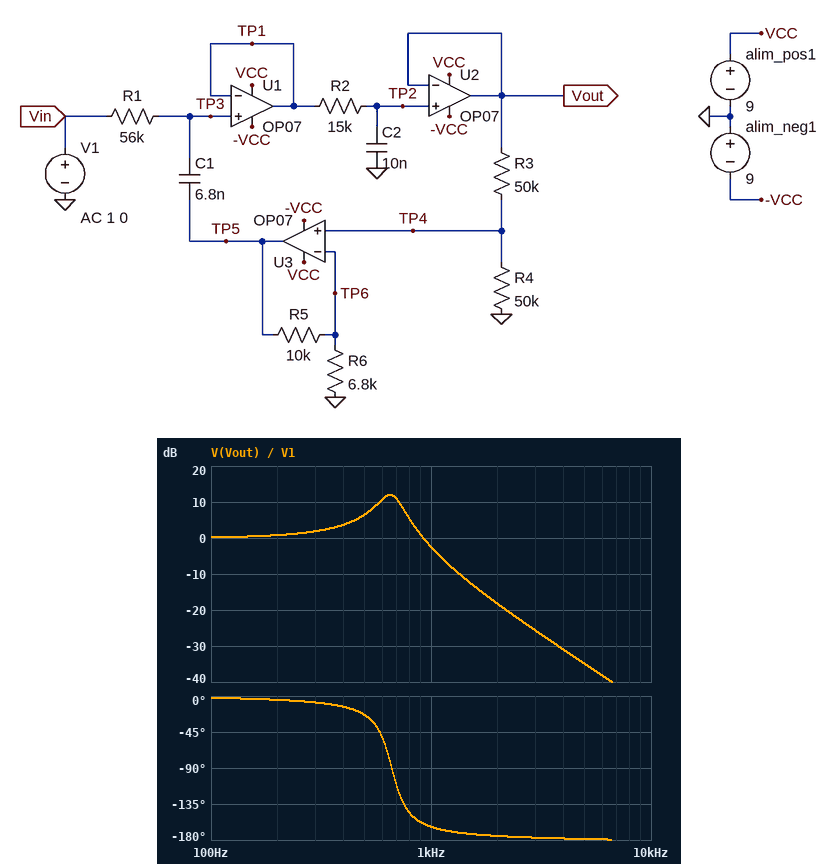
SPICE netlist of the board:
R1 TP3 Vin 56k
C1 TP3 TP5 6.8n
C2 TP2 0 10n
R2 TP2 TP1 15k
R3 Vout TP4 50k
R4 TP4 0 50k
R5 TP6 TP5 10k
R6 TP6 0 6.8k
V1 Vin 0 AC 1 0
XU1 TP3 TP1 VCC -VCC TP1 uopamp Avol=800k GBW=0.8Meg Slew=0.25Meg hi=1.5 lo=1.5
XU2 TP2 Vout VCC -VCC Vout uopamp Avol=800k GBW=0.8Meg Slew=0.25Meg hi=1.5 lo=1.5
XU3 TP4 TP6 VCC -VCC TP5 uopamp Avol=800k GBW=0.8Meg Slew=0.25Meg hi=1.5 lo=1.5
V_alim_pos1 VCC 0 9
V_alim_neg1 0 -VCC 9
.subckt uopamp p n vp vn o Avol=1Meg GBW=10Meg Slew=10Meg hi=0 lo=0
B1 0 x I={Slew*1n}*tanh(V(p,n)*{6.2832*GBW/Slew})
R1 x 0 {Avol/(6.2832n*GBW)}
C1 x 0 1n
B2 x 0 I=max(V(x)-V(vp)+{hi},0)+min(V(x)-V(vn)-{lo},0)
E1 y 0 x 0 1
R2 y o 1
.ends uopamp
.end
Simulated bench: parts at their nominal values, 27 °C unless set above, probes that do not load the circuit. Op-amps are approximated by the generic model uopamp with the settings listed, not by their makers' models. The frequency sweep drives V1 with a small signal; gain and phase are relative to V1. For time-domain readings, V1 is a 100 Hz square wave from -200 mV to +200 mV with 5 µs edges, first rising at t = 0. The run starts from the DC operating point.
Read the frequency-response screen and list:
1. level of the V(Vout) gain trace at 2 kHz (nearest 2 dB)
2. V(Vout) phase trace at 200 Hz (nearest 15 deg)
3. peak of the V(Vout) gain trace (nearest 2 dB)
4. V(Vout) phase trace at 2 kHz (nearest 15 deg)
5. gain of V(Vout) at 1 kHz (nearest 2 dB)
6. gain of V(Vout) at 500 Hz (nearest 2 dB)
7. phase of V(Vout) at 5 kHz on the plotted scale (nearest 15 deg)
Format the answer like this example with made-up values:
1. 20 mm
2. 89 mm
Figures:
1. -18 dB
2. 0 deg
3. 12 dB
4. -180 deg
5. -2 dB
6. 6 dB
7. -180 deg
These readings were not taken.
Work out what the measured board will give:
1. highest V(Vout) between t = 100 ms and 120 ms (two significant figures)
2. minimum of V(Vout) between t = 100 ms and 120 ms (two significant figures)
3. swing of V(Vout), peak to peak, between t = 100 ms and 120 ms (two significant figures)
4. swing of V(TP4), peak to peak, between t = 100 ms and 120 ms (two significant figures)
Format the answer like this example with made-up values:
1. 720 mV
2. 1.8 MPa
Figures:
1. 470 mV
2. -470 mV
3. 940 mV
4. 470 mV
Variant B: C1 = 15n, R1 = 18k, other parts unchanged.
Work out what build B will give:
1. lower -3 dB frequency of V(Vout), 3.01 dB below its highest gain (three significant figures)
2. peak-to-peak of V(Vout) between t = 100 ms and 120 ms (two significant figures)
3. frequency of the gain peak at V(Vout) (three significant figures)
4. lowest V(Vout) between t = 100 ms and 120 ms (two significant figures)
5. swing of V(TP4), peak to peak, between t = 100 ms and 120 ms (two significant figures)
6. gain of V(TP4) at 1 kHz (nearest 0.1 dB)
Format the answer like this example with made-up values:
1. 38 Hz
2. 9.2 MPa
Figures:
1. 552 Hz
2. 800 mV
3. 751 Hz
4. -400 mV
5. 400 mV
6. -4.3 dB
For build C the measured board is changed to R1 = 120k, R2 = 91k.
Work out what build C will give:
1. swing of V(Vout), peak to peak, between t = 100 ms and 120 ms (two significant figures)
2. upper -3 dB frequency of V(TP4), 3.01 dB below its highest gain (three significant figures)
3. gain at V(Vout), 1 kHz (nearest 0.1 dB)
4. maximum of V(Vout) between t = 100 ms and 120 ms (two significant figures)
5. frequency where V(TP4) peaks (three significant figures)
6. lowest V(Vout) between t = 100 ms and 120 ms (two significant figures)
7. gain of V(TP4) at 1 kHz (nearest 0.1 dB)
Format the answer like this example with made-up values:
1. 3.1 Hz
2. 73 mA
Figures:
1. 590 mV
2. 219 Hz
3. -29.2 dB
4. 290 mV
5. 149 Hz
6. -290 mV
7. -35.2 dB
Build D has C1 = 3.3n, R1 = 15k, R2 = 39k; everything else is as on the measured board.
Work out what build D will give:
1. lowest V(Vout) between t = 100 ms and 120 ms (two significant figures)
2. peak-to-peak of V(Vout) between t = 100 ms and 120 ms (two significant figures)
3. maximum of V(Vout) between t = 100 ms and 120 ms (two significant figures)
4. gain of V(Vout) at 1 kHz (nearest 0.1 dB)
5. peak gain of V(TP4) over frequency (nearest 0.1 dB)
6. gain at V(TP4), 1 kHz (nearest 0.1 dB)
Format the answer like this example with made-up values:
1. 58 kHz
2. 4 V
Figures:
1. -200 mV
2. 400 mV
3. 200 mV
4. -7.6 dB
5. -6.0 dB
6. -13.6 dB
